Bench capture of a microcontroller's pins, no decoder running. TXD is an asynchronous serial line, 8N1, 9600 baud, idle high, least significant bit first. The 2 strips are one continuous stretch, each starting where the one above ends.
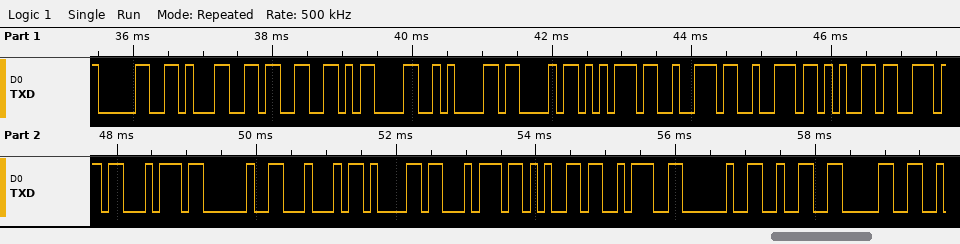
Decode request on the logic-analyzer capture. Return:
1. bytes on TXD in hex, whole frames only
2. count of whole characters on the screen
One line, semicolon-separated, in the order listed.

30 31 33 0D 0A 43 75 72 72 65 6E 74 20 44 61 74 65 3A 20 32 30; 21
